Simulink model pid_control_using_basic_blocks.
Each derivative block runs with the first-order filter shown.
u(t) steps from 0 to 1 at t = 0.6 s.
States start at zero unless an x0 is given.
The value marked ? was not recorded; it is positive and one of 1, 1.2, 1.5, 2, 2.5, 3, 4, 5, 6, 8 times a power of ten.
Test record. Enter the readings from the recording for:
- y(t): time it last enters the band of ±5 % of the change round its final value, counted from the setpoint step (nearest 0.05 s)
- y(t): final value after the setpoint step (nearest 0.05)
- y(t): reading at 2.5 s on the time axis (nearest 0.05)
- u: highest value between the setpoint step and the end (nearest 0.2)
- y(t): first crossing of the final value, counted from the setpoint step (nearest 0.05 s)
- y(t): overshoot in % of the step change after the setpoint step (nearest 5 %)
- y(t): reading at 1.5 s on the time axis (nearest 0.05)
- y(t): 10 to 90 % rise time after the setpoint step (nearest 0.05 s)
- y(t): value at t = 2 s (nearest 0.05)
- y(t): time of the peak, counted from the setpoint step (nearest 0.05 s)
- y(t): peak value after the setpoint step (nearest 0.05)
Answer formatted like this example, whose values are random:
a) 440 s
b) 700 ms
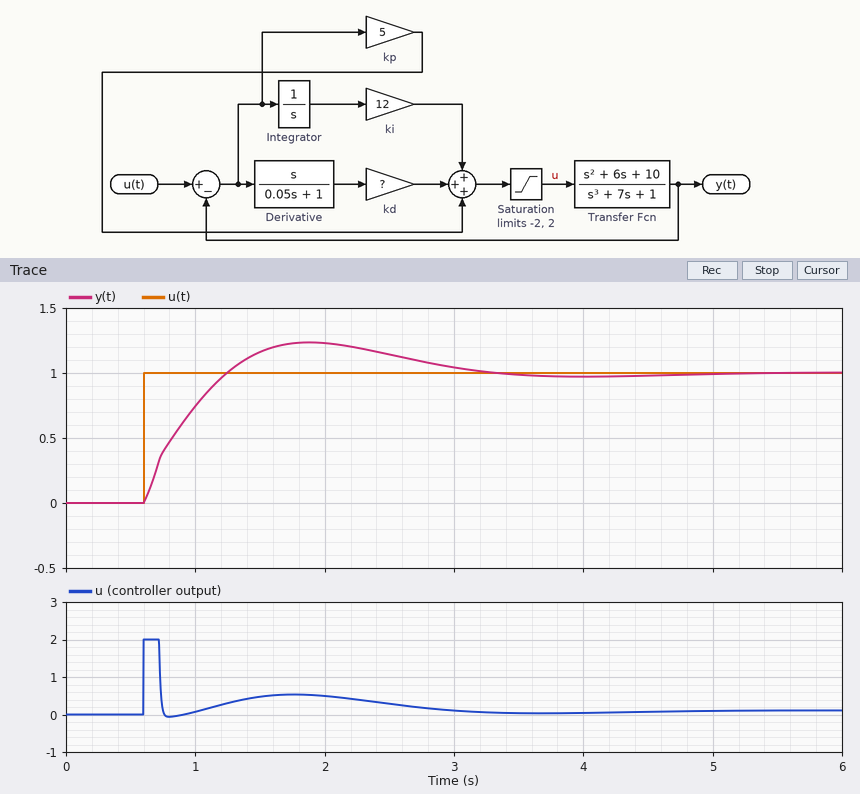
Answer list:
a) 2.35 s
b) 1.00
c) 1.15
d) 2.0
e) 0.65 s
f) 25 %
g) 1.15
h) 0.50 s
i) 1.25
j) 1.30 s
k) 1.25
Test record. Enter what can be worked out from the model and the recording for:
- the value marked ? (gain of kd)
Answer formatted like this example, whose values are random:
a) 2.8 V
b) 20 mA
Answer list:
a) 3
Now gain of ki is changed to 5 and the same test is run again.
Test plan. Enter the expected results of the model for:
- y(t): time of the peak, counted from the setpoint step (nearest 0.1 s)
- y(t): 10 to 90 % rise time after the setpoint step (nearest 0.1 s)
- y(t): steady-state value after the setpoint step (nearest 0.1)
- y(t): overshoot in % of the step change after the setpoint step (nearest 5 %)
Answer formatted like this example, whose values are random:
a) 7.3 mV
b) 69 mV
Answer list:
a) 2.1 s
b) 0.7 s
c) 1.0
d) 15 %
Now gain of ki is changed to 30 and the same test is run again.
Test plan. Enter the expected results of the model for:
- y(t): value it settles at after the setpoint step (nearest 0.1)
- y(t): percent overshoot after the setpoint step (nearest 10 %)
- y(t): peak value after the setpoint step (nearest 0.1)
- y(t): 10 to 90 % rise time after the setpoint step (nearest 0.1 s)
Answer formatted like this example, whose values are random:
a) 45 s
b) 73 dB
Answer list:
a) 1.0
b) 40 %
c) 1.4
d) 0.3 s
